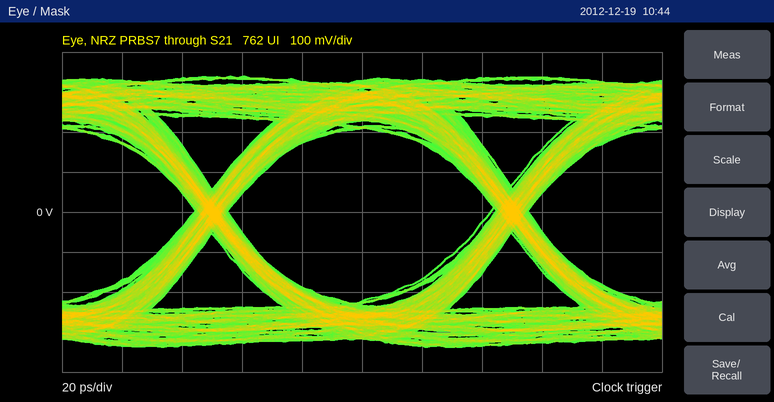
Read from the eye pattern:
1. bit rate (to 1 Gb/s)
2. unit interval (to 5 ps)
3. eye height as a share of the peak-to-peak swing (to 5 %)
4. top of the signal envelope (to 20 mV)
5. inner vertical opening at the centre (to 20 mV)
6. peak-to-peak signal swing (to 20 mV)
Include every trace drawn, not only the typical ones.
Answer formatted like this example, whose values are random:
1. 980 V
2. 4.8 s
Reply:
1. 10 Gb/s
2. 100 ps
3. 65 %
4. 340 mV
5. 440 mV
6. 680 mV
